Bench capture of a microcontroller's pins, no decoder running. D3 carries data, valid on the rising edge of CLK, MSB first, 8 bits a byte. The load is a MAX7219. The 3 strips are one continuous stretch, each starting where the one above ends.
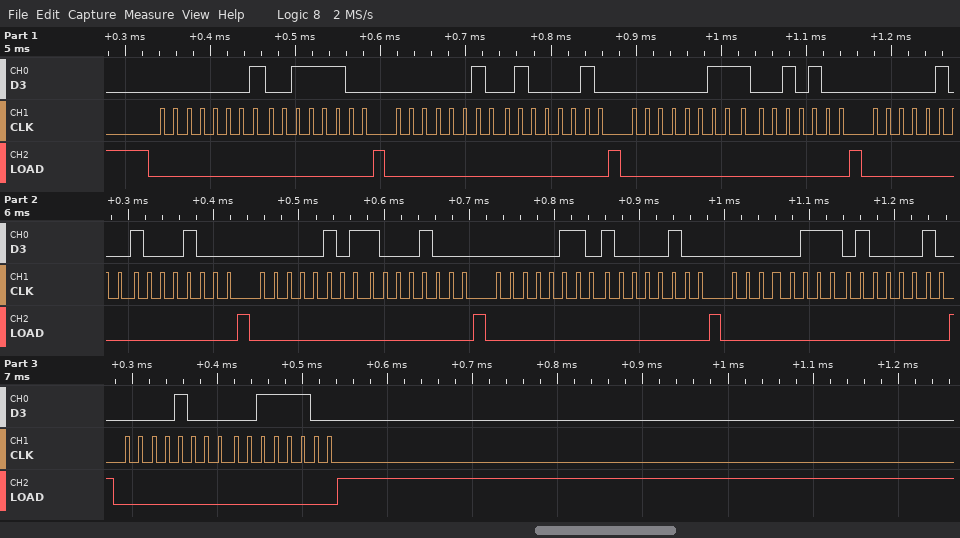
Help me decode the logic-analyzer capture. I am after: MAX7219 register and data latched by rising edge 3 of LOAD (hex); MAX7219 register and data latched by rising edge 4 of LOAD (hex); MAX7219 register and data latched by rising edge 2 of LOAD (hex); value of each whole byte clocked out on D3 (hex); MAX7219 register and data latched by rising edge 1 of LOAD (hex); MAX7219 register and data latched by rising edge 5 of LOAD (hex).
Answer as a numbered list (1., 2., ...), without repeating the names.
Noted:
1. register 0x3, data 0x94
2. register 0x4, data 0x88
3. register 0x2, data 0x42
4. 01 3C 02 42 03 94 04 88 05 88 06 84 07 42 08 3C
5. register 0x1, data 0x3C
6. register 0x5, data 0x88
